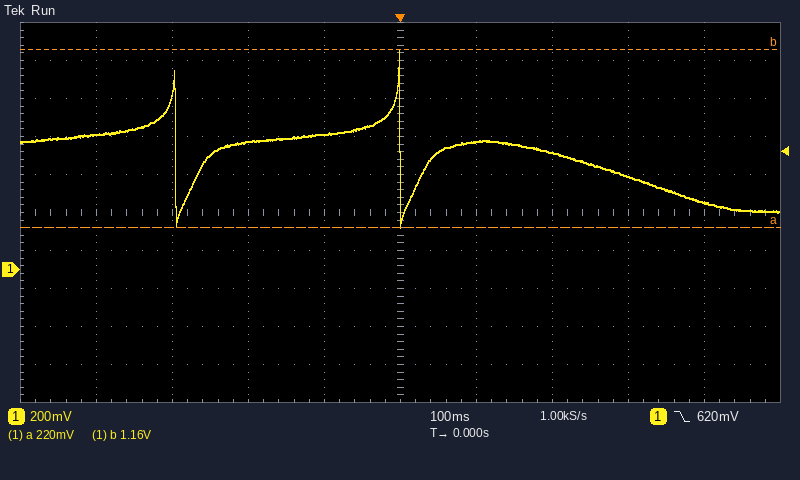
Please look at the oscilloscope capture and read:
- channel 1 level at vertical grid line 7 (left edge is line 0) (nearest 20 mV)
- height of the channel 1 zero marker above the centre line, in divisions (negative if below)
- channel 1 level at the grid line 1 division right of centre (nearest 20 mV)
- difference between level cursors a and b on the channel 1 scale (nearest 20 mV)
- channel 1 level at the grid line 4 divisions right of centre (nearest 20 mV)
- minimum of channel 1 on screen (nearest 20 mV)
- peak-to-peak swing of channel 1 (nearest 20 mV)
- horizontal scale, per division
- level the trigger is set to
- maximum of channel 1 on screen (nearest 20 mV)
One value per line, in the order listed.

620 mV
-1.5 div
680 mV
940 mV
360 mV
220 mV
940 mV
100 ms
620 mV
1.16 V
